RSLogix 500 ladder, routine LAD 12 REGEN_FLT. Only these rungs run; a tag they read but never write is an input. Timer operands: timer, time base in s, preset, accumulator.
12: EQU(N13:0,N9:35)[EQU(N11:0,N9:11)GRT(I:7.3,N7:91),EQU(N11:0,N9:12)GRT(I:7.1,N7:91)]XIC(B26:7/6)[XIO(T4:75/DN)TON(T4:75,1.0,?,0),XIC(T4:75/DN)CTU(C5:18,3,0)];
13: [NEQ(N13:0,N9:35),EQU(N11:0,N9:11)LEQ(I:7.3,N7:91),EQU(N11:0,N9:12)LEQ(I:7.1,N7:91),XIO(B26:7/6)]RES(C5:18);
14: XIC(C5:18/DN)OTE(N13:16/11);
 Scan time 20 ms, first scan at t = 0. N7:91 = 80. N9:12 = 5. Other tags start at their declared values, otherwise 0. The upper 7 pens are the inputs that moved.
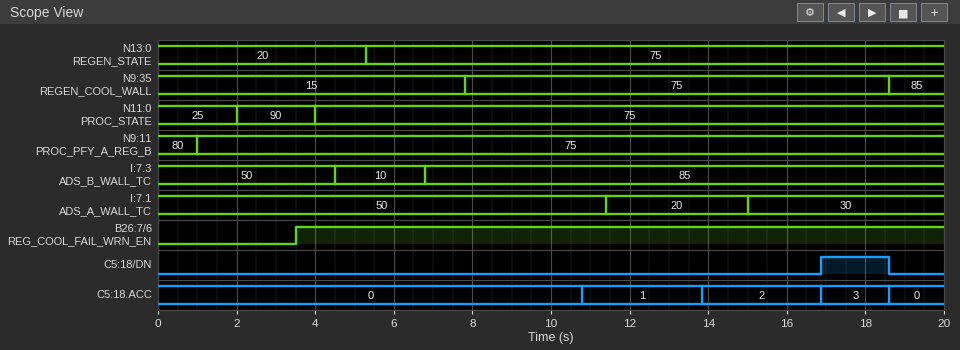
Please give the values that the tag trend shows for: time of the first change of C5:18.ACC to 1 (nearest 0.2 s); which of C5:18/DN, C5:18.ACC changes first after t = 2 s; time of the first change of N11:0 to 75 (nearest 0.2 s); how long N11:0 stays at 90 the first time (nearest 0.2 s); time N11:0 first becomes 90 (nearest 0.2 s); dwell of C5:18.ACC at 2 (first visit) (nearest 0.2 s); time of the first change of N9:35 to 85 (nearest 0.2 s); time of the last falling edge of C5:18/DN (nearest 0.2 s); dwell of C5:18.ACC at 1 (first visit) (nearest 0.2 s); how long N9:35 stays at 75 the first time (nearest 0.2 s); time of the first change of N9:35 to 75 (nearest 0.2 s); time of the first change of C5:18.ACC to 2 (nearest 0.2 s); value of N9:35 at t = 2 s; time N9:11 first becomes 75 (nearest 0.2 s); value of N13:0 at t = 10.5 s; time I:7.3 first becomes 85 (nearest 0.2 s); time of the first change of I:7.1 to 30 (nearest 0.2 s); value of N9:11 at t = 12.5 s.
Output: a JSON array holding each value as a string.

["10.8 s", "C5:18.ACC", "4.0 s", "2.0 s", "2.0 s", "3.0 s", "18.6 s", "18.6 s", "3.0 s", "10.8 s", "7.8 s", "13.8 s", "15", "1.0 s", "75", "6.8 s", "15.0 s", "75"]
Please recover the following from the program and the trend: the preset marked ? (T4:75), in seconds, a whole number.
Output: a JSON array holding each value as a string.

["3 s"]
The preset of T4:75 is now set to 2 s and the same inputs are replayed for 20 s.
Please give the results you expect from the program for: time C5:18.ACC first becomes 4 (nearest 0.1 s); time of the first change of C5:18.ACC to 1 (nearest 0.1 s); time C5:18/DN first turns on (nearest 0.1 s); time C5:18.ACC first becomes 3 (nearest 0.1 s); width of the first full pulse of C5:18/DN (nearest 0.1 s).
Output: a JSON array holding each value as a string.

["15.9 s", "9.8 s", "13.9 s", "13.9 s", "4.7 s"]
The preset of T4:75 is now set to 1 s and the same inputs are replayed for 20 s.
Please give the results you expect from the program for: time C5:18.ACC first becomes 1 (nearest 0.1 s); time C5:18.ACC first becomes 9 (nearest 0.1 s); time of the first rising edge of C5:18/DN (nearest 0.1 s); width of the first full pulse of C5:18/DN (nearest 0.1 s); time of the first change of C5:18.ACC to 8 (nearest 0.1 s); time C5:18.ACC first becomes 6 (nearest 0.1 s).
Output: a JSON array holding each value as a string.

["8.8 s", "17.1 s", "10.9 s", "7.7 s", "16.1 s", "14.0 s"]
